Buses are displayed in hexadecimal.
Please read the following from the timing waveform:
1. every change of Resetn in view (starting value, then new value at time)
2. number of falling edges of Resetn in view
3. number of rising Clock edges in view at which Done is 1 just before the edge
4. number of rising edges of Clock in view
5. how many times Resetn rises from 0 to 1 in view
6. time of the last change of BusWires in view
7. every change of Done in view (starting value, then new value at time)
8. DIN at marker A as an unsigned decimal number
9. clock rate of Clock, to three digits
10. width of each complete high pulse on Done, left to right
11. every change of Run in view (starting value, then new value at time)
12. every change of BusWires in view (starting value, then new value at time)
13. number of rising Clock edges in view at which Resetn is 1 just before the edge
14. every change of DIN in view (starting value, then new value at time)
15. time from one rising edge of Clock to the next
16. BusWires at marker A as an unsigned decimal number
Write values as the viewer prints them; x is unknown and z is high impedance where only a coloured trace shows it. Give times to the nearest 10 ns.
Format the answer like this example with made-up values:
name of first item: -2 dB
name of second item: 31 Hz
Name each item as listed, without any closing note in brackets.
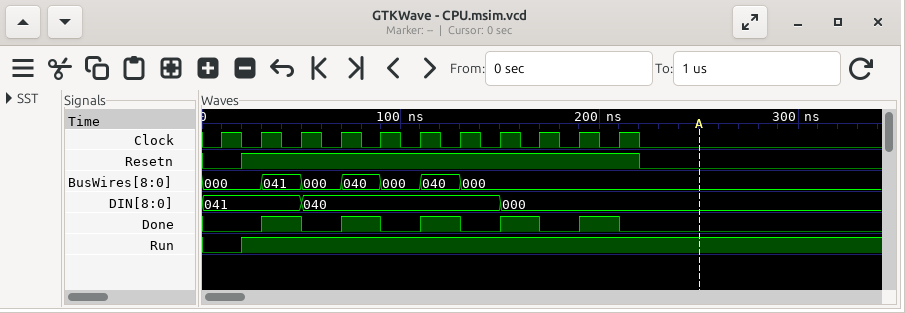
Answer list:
every change of Resetn in view: 0, 1 at 20 ns, 0 at 220 ns
number of falling edges of Resetn in view: 1
number of rising Clock edges in view at which Done is 1 just before the edge: 5
number of rising edges of Clock in view: 11
how many times Resetn rises from 0 to 1 in view: 1
time of the last change of BusWires in view: 130 ns
every change of Done in view: 0, 1 at 30 ns, 0 at 50 ns, 1 at 70 ns, 0 at 90 ns, 1 at 110 ns, 0 at 130 ns, 1 at 150 ns, 0 at 170 ns, 1 at 190 ns, 0 at 210 ns
DIN at marker A as an unsigned decimal number: 0
clock rate of Clock, to three digits: 50.0 MHz
width of each complete high pulse on Done, left to right: 20 ns, 20 ns, 20 ns, 20 ns, 20 ns
every change of Run in view: 0, 1 at 20 ns
every change of BusWires in view: 000, 041 at 30 ns, 000 at 50 ns, 040 at 70 ns, 000 at 90 ns, 040 at 110 ns, 000 at 130 ns
number of rising Clock edges in view at which Resetn is 1 just before the edge: 10
every change of DIN in view: 041, 040 at 50 ns, 000 at 150 ns
time from one rising edge of Clock to the next: 20 ns
BusWires at marker A as an unsigned decimal number: 0
